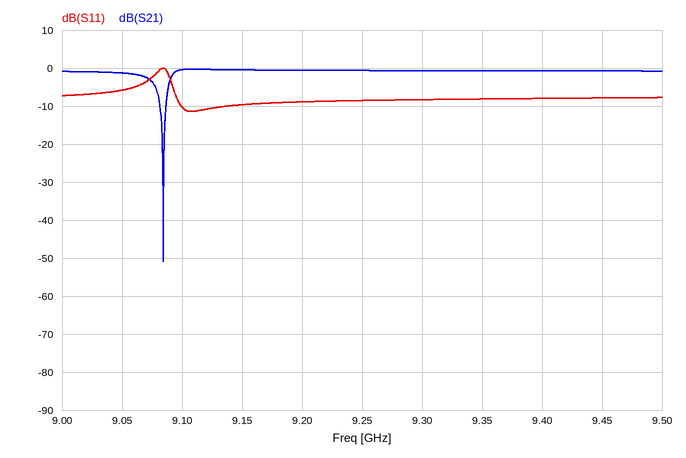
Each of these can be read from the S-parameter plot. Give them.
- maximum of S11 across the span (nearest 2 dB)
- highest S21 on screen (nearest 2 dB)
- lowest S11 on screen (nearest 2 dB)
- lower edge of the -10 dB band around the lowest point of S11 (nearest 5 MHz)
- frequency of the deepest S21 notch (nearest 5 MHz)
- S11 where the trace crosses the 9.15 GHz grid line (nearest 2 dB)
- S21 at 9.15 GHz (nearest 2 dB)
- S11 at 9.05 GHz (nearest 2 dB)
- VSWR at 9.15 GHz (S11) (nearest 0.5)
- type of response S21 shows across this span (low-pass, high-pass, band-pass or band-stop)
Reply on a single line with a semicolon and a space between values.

0 dB; 0 dB; -12 dB; 9.100 GHz; 9.085 GHz; -10 dB; 0 dB; -6 dB; 2.0; band-stop
